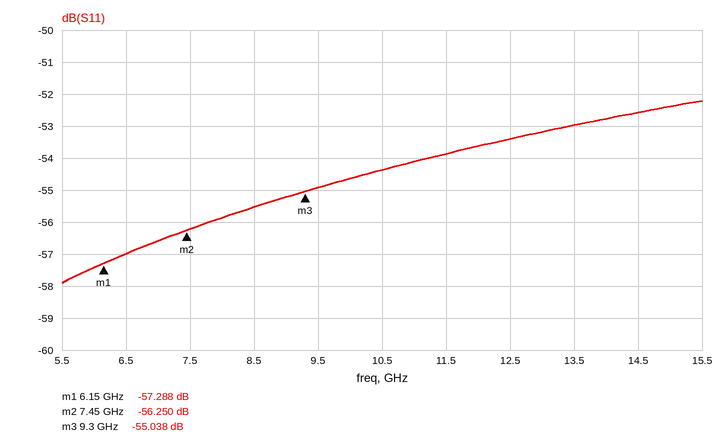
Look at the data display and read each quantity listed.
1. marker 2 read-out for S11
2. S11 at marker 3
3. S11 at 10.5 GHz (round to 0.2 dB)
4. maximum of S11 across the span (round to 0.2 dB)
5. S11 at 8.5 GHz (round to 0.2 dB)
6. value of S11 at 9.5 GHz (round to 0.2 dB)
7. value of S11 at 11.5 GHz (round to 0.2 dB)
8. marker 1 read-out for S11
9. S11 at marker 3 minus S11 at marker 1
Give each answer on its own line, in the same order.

-56.250 dB
-55.038 dB
-54.4 dB
-52.2 dB
-55.6 dB
-55.0 dB
-53.8 dB
-57.288 dB
2.250 dB
